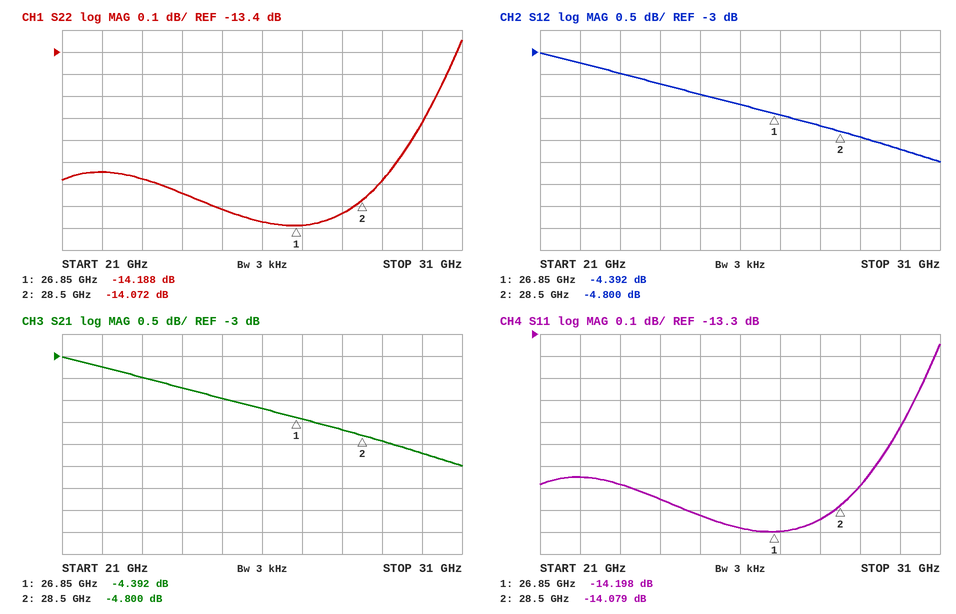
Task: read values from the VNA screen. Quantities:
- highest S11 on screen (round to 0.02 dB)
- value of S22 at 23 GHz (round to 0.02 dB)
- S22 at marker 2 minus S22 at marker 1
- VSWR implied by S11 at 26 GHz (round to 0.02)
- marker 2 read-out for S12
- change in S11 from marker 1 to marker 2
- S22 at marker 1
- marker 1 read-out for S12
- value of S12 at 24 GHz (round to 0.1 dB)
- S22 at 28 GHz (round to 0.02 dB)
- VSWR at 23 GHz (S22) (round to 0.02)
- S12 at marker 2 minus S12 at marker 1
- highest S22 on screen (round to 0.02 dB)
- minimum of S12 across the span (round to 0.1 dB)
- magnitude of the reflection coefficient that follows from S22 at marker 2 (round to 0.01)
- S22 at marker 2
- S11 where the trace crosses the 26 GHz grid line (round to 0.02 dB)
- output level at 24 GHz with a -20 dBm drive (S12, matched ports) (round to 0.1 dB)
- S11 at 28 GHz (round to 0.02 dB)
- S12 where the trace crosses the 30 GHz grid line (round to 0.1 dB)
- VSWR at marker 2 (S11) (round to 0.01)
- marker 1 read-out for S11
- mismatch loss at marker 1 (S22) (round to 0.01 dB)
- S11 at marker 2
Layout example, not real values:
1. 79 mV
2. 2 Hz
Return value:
1. -13.34 dB
2. -13.98 dB
3. 0.116 dB
4. 1.48
5. -4.800 dB
6. 0.119 dB
7. -14.188 dB
8. -4.392 dB
9. -3.7 dB
10. -14.14 dB
11. 1.50
12. -0.408 dB
13. -13.34 dB
14. -5.5 dB
15. 0.20
16. -14.072 dB
17. -14.18 dB
18. -23.7 dBm
19. -14.14 dB
20. -5.2 dB
21. 1.49
22. -14.198 dB
23. 0.17 dB
24. -14.079 dB
